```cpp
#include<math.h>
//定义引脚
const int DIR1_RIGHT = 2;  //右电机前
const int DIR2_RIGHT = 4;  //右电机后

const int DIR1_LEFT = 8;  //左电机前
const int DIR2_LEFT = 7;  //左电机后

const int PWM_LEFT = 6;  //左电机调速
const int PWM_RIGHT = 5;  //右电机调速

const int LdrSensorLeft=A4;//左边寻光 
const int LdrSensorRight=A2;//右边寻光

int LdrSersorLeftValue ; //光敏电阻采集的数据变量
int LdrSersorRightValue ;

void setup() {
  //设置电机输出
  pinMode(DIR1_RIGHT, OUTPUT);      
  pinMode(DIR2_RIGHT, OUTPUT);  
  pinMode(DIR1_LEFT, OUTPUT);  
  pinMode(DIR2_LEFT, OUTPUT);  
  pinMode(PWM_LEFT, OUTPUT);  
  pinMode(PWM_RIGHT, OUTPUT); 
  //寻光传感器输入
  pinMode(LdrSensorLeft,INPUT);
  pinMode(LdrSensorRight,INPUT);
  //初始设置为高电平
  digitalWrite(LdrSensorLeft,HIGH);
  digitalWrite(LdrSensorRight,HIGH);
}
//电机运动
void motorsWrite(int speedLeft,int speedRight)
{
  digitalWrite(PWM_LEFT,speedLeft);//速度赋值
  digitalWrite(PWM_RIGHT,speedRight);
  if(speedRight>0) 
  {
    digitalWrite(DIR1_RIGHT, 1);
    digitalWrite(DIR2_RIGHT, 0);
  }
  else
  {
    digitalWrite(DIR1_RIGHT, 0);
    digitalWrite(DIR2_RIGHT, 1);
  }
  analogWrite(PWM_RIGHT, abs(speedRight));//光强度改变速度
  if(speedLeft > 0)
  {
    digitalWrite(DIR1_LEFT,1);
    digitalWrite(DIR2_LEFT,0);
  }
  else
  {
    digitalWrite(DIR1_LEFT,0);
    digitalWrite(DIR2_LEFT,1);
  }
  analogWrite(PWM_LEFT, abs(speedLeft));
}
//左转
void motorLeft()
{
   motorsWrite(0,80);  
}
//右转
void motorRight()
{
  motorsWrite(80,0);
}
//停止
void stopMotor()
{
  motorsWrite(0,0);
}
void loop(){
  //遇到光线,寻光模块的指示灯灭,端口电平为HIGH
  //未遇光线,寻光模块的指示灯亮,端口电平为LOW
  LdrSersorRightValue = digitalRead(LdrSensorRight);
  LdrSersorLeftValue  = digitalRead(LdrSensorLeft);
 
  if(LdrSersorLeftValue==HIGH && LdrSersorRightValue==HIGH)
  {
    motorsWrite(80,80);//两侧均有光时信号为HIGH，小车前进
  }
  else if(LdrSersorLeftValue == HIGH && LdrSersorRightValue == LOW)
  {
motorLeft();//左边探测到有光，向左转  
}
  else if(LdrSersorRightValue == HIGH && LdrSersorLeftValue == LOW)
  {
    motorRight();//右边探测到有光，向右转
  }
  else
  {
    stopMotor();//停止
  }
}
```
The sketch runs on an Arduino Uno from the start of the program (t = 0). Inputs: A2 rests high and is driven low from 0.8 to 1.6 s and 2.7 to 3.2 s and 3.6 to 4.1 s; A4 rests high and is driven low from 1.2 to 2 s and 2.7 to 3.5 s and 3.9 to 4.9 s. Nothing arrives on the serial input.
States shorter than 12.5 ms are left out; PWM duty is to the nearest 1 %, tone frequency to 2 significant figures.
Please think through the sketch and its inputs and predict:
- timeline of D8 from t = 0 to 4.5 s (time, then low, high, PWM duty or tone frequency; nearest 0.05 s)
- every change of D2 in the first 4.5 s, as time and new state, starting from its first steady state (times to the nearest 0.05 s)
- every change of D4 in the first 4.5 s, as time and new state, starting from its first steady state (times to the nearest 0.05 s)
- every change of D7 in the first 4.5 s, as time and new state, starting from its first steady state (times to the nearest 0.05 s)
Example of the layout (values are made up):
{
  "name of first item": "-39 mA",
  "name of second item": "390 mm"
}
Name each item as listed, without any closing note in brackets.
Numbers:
{
  "timeline of D8 from t = 0 to 4.5 s": "0 s high; 0.8 s low; 1.6 s high; 2.7 s low; 3.2 s high; 3.6 s low; 4.1 s high",
  "every change of D2 in the first 4.5 s, as time and new state, starting from its first steady state": "0 s high; 1.2 s low; 2 s high; 2.7 s low; 3.5 s high; 3.9 s low",
  "every change of D4 in the first 4.5 s, as time and new state, starting from its first steady state": "0 s low; 1.2 s high; 2 s low; 2.7 s high; 3.5 s low; 3.9 s high",
  "every change of D7 in the first 4.5 s, as time and new state, starting from its first steady state": "0 s low; 0.8 s high; 1.6 s low; 2.7 s high; 3.2 s low; 3.6 s high; 4.1 s low"
}
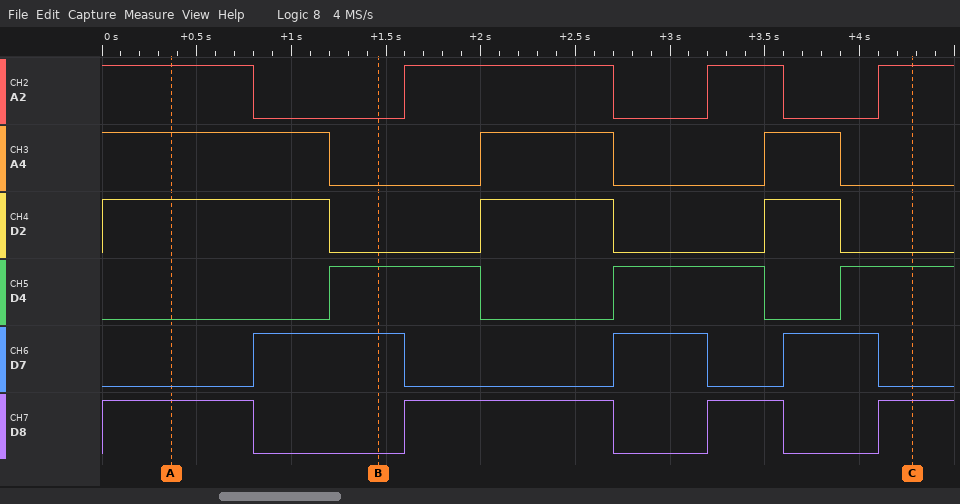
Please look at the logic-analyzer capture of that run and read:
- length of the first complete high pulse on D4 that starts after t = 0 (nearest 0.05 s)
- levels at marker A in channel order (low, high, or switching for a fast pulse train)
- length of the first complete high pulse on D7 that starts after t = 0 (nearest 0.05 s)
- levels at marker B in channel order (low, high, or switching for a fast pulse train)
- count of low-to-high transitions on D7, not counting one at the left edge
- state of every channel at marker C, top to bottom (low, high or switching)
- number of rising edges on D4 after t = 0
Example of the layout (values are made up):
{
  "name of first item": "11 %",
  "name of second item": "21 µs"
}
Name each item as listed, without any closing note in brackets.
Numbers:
{
  "length of the first complete high pulse on D4 that starts after t = 0": "0.80 s",
  "levels at marker A in channel order": "A2 high, A4 high, D2 high, D4 low, D7 low, D8 high",
  "length of the first complete high pulse on D7 that starts after t = 0": "0.80 s",
  "levels at marker B in channel order": "A2 low, A4 low, D2 low, D4 high, D7 high, D8 low",
  "count of low-to-high transitions on D7, not counting one at the left edge": "3",
  "state of every channel at marker C, top to bottom": "A2 high, A4 low, D2 low, D4 high, D7 low, D8 high",
  "number of rising edges on D4 after t = 0": "3"
}
